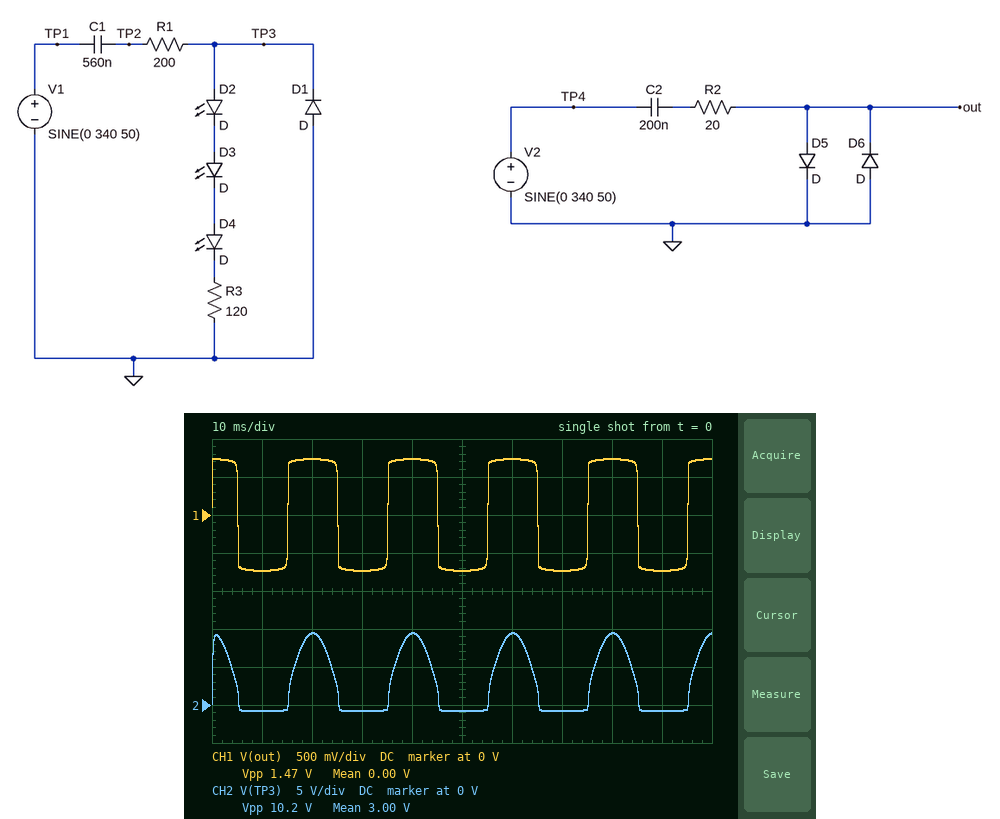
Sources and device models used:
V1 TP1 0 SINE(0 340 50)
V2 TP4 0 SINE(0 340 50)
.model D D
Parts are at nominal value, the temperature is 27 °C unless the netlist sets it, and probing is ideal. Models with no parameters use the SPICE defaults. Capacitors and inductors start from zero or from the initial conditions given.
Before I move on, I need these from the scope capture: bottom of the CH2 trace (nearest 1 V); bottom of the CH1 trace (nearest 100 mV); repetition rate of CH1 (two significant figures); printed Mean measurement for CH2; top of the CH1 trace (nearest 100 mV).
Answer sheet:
-1 V
-700 mV
50 Hz
3.00 V
700 mV
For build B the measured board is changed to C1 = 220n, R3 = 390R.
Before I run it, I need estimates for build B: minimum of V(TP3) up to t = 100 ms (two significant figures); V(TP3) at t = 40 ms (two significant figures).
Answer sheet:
-740 mV
11 V
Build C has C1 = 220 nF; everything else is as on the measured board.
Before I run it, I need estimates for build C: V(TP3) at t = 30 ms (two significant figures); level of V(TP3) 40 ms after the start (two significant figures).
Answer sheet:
-740 mV
5.0 V
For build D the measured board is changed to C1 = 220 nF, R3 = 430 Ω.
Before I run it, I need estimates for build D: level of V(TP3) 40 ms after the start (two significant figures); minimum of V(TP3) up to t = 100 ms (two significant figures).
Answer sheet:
12 V
-740 mV
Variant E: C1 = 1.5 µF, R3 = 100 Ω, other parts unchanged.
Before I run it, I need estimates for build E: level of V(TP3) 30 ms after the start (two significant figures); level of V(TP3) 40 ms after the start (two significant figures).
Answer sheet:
-790 mV
18 V
